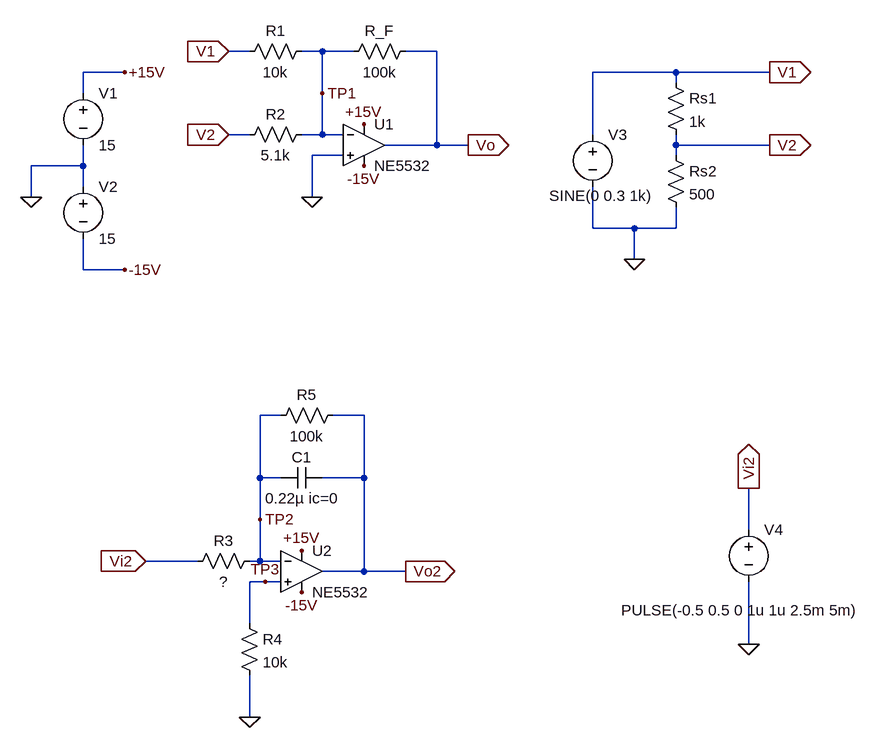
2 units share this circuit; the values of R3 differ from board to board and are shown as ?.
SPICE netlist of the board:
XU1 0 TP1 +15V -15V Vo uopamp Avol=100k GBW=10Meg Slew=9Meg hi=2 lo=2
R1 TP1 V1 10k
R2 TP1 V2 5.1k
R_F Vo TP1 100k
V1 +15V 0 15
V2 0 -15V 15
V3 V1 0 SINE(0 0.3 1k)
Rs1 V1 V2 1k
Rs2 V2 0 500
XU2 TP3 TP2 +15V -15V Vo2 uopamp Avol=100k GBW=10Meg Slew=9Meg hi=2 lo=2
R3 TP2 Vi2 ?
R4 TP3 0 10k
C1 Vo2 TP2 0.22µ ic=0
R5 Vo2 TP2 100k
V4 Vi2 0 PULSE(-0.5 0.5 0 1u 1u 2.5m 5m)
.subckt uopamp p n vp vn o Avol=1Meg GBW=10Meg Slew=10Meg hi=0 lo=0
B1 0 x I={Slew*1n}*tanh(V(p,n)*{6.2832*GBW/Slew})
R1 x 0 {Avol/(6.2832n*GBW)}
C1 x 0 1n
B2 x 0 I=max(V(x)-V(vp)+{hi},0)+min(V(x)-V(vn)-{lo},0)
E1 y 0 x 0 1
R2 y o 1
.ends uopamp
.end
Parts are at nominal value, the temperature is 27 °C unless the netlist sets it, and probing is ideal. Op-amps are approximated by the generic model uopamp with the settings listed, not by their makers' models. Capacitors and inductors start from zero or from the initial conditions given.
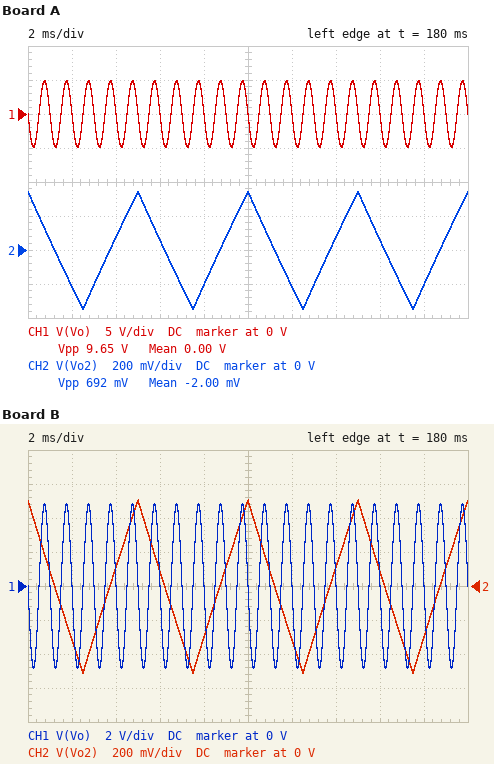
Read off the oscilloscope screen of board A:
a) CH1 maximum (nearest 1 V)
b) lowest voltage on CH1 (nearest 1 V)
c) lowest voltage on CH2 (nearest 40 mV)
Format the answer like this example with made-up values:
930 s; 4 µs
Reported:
5 V; -5 V; -360 mV
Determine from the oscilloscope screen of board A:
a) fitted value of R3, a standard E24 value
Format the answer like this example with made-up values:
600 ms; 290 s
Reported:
8.2 kΩ
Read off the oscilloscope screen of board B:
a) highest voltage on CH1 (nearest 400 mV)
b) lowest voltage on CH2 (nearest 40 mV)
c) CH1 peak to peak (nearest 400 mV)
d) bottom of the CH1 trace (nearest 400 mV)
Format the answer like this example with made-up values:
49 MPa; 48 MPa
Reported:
4.8 V; -520 mV; 9.6 V; -4.8 V
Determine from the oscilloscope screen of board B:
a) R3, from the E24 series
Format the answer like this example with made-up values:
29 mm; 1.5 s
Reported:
5.6 kΩ
